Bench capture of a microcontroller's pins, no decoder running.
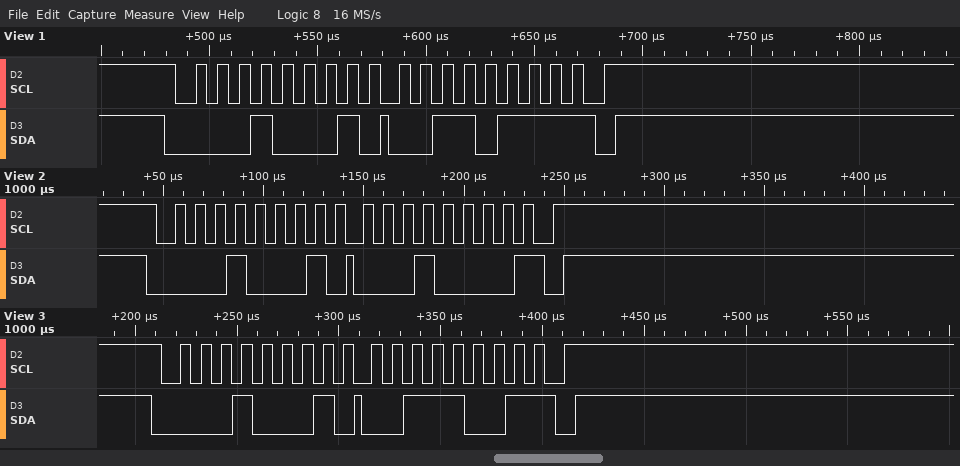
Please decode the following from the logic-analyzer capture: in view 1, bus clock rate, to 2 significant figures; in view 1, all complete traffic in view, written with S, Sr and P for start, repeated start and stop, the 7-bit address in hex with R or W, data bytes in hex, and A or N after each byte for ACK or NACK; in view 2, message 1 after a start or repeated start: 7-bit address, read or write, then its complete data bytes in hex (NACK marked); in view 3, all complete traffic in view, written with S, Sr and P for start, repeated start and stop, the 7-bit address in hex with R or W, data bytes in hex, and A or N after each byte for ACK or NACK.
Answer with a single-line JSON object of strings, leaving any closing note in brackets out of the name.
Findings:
{"in view 1, bus clock rate, to 2 significant figures": "100 kHz", "in view 1, all complete traffic in view, written with S, Sr and P for start, repeated start and stop, the 7-bit address in hex with R or W, data bytes in hex, and A or N after each byte for ACK or NACK": "S 08R A 37 N P", "in view 2, message 1 after a start or repeated start: 7-bit address, read or write, then its complete data bytes in hex": "0x08 read: 10 NACK", "in view 3, all complete traffic in view, written with S, Sr and P for start, repeated start and stop, the 7-bit address in hex with R or W, data bytes in hex, and A or N after each byte for ACK or NACK": "S 08R A 39 N P"}
